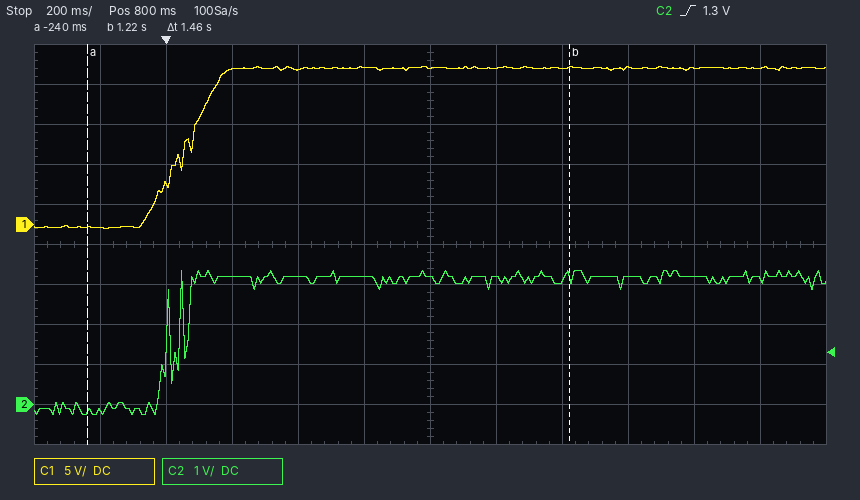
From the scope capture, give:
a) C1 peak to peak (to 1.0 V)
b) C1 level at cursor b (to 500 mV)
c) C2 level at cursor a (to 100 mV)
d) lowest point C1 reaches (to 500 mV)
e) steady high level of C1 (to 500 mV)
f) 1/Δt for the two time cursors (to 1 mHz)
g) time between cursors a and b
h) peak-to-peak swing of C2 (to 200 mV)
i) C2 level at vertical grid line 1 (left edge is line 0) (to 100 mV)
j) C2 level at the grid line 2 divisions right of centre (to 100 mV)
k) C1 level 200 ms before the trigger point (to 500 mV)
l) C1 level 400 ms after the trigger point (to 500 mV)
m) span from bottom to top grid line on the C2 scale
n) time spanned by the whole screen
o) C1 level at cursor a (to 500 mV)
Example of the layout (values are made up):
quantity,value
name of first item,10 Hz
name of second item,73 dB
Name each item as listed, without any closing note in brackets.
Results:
quantity,value
C1 peak to peak,20.0 V
C1 level at cursor b,19.5 V
C2 level at cursor a,-200 mV
lowest point C1 reaches,-500 mV
steady high level of C1,19.5 V
1/Δt for the two time cursors,685 mHz
time between cursors a and b,1.46 s
peak-to-peak swing of C2,3.6 V
C2 level at vertical grid line 1 (left edge is line 0),-200 mV
C2 level at the grid line 2 divisions right of centre,3.1 V
C1 level 200 ms before the trigger point,-500 mV
C1 level 400 ms after the trigger point,19.5 V
span from bottom to top grid line on the C2 scale,10 V
time spanned by the whole screen,2.4 s
C1 level at cursor a,-500 mV
